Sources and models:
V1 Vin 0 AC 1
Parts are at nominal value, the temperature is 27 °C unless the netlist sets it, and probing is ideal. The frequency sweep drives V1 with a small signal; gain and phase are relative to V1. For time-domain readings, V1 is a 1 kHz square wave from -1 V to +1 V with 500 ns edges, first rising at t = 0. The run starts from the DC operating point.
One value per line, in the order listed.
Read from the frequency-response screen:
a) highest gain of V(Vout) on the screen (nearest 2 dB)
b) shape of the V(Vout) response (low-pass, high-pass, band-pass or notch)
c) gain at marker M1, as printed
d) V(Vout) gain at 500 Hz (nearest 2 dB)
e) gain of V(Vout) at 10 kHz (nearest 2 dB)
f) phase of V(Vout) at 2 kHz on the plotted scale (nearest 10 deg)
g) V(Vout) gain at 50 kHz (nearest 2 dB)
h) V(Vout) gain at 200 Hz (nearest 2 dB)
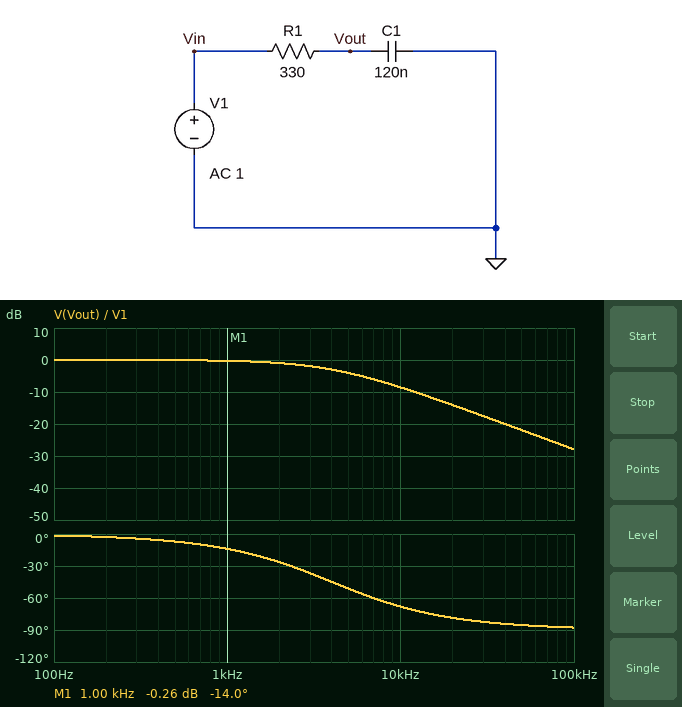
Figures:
0 dB
low-pass
-0.26 dB
0 dB
-8 dB
-30 deg
-22 dB
0 dB
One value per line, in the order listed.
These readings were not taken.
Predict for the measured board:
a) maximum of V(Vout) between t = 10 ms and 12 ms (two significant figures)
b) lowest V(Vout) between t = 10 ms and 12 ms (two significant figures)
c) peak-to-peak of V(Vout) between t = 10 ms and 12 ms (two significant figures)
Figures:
1.0 V
-1.0 V
2.0 V
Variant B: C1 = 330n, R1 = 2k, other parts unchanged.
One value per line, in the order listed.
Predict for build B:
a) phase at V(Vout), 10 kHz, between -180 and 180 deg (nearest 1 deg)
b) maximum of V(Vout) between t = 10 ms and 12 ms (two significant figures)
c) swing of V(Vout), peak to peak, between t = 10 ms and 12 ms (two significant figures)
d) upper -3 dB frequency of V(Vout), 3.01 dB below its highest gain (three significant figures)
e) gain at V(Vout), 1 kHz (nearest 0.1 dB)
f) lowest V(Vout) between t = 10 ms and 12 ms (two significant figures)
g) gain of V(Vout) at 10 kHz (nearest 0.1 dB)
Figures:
-89 deg
360 mV
720 mV
241 Hz
-12.6 dB
-360 mV
-32.4 dB
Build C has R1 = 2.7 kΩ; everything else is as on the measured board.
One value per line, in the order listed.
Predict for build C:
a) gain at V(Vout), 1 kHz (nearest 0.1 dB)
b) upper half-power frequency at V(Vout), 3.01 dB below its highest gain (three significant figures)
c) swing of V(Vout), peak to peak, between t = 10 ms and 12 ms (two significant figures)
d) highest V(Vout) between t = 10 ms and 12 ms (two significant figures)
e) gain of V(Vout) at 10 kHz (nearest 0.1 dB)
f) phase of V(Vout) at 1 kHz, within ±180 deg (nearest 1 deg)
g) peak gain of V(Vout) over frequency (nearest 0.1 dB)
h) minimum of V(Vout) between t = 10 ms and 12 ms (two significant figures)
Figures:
-7.1 dB
491 Hz
1.3 V
650 mV
-26.2 dB
-64 deg
0 dB
-650 mV
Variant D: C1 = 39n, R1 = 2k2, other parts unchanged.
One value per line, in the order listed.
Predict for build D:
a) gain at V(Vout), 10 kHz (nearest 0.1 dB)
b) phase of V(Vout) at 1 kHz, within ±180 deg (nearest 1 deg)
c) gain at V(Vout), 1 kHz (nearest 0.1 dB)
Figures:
-14.8 dB
-28 deg
-1.1 dB
